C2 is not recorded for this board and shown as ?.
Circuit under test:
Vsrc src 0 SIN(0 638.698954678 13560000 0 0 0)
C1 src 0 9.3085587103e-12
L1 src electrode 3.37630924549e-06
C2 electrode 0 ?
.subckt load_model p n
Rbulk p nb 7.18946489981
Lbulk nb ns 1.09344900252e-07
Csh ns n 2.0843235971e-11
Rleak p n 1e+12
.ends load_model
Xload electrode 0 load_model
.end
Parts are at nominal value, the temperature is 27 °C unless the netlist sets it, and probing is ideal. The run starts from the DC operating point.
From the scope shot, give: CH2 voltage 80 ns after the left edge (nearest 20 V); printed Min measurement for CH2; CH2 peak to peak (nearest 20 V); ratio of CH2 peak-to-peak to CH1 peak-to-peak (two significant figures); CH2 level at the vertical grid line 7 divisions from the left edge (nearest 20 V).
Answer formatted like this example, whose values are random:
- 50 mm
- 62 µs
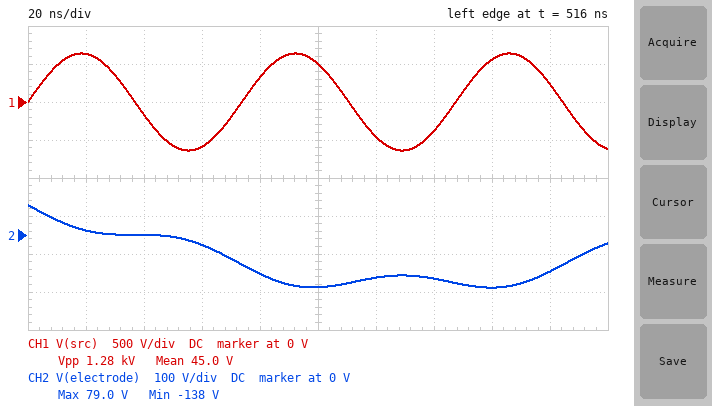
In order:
- -100 V
- -138 V
- 220 V
- 0.17
- -120 V
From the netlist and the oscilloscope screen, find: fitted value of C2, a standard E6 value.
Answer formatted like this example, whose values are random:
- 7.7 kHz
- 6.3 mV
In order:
- 1 nF
